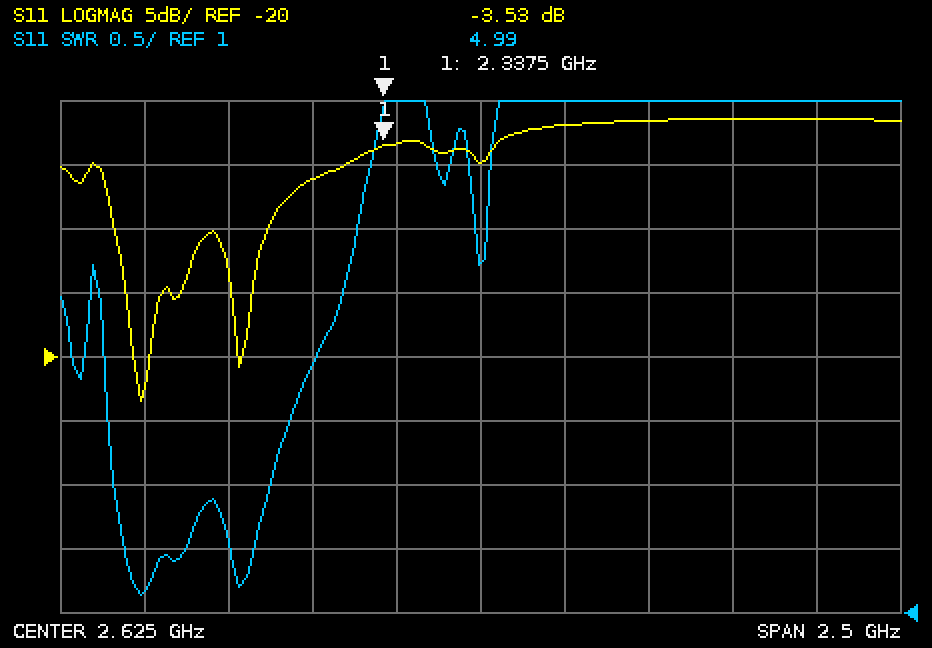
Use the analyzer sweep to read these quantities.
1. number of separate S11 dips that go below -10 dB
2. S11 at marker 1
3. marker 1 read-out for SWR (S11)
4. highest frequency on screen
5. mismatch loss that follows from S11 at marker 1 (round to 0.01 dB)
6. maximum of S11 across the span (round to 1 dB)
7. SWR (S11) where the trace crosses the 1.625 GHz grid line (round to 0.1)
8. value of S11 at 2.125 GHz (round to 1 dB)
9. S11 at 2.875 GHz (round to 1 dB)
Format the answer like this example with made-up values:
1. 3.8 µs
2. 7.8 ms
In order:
1. 2
2. -3.53 dB
3. 4.99
4. 3.875 GHz
5. 2.55 dB
6. -1 dB
7. 1.2
8. -6 dB
9. -2 dB
